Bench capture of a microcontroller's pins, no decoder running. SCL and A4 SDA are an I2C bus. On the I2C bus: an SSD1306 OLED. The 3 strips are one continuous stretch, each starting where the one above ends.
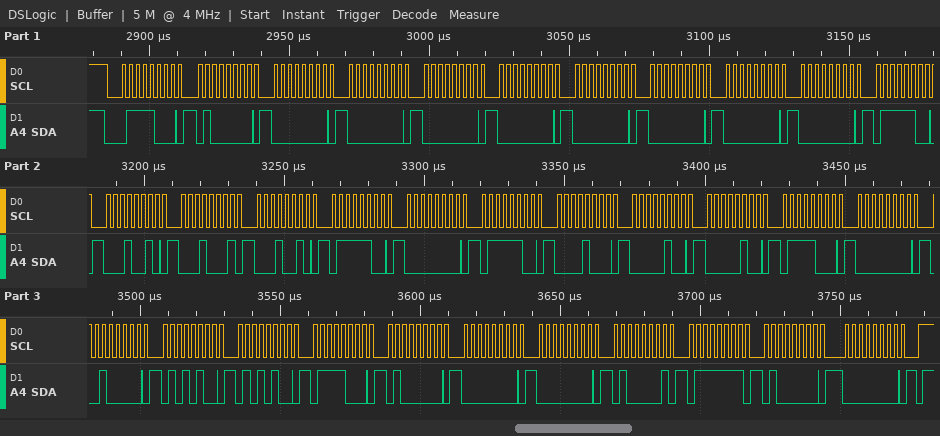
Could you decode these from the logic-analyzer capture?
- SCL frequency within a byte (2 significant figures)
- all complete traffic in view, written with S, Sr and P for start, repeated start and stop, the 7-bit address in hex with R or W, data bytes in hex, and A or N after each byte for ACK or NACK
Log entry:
400 kHz
S 3CW A 40 A 00 A 00 A 00 A 00 A 00 A 00 A 00 A 00 A 7C A 12 A 11 A 12 A 7C A 00 A 7C A 08 A 04 A 04 A 78 A 00 A 20 A 54 A 54 A 78 A 40 A 00 A 00 A 41 A 7F A 40 A 00 A P
